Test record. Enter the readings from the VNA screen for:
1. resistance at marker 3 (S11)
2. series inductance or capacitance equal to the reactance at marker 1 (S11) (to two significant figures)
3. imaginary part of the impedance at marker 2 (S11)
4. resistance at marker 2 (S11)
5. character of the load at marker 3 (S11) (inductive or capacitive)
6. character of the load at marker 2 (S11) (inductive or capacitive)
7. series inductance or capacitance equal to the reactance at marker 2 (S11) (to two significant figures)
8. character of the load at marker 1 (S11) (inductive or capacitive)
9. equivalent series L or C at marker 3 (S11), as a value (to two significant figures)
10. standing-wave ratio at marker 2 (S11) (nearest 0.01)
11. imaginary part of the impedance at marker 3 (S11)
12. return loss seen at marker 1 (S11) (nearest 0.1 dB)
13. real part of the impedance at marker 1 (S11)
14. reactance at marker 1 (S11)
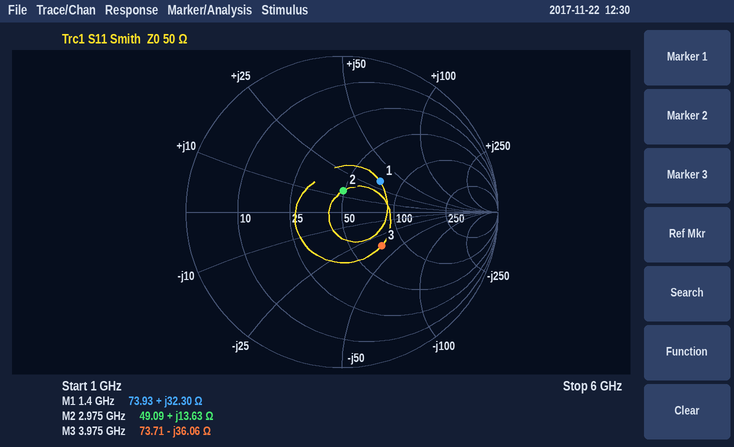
73.71 Ω
3.7 nH
+13.63 Ω
49.09 Ω
capacitive
inductive
730 pH
inductive
1.1 pF
1.32
-36.06 Ω
10.1 dB
73.93 Ω
+32.30 Ω
